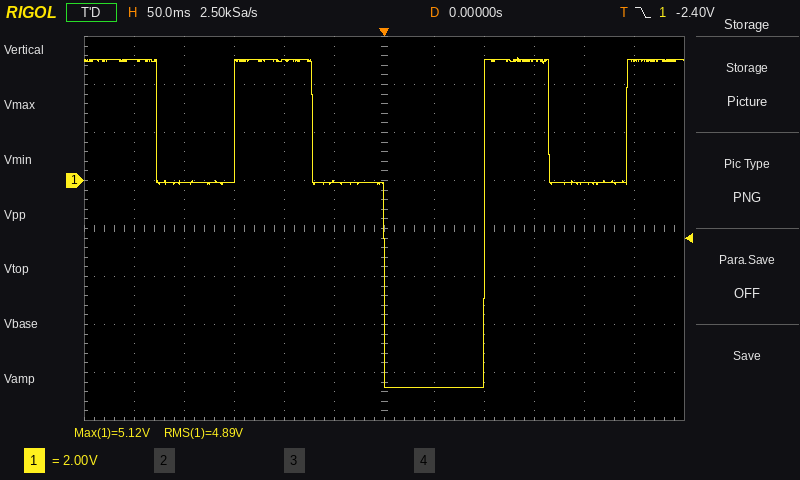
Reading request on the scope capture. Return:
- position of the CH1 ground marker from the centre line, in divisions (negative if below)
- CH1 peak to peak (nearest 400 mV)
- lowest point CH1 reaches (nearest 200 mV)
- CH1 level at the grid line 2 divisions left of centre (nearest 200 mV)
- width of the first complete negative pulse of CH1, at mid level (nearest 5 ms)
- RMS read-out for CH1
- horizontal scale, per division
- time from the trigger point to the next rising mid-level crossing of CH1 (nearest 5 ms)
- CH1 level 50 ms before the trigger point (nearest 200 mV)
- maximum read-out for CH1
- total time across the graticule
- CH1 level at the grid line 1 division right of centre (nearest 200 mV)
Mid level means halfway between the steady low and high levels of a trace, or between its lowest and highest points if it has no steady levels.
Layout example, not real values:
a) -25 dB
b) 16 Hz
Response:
a) +1.0 div
b) 13.6 V
c) -8.6 V
d) 5.0 V
e) 100 ms
f) 4.89 V
g) 50 ms
h) 100 ms
i) 0.0 V
j) 5.12 V
k) 600 ms
l) -8.6 V
